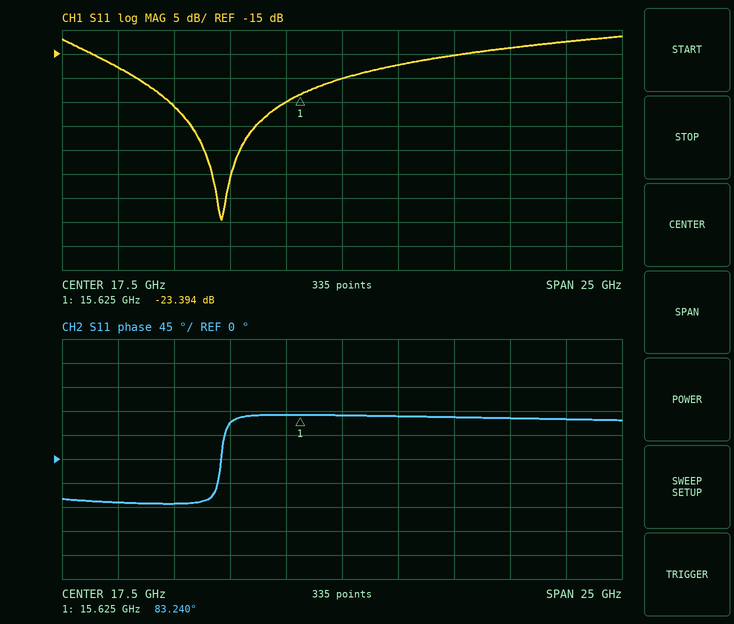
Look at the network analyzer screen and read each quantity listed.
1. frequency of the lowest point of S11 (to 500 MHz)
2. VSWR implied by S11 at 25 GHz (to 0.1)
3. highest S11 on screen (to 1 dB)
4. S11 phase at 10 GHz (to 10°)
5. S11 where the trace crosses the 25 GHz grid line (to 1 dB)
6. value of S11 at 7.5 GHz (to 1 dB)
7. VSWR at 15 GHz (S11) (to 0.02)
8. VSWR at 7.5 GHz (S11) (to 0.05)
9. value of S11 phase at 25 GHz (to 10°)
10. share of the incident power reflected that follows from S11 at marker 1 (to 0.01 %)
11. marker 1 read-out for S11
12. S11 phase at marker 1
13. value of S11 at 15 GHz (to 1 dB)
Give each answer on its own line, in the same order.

12.0 GHz
1.5
-11 dB
-80°
-14 dB
-18 dB
1.12
1.30
80°
0.46 %
-23.394 dB
83.240°
-25 dB
